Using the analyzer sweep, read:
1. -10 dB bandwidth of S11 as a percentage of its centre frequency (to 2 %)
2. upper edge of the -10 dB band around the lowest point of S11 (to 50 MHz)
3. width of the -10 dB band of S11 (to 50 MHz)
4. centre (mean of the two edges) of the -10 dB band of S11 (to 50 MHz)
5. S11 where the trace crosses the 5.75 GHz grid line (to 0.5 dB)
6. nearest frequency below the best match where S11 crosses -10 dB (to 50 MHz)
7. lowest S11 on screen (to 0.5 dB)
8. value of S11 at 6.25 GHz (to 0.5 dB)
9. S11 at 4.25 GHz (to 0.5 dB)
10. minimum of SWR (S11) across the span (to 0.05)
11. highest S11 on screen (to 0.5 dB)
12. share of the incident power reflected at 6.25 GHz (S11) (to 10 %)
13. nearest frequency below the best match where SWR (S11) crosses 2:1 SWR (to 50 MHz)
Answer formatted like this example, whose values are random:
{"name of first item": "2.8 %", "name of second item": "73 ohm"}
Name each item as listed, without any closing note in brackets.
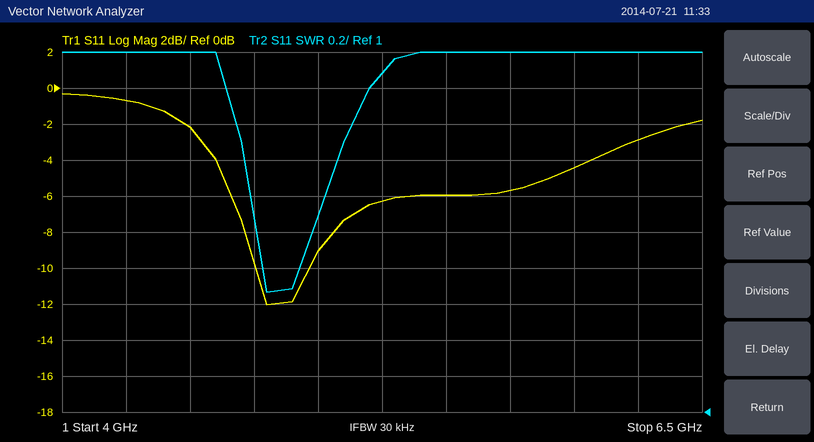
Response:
{"-10 dB bandwidth of S11 as a percentage of its centre frequency": "4 %", "upper edge of the -10 dB band around the lowest point of S11": "4.95 GHz", "width of the -10 dB band of S11": "200 MHz", "centre (mean of the two edges) of the -10 dB band of S11": "4.85 GHz", "S11 where the trace crosses the 5.75 GHz grid line": "-5.5 dB", "nearest frequency below the best match where S11 crosses -10 dB": "4.75 GHz", "lowest S11 on screen": "-12.0 dB", "value of S11 at 6.25 GHz": "-3.0 dB", "S11 at 4.25 GHz": "-0.5 dB", "minimum of SWR (S11) across the span": "1.65", "highest S11 on screen": "-0.5 dB", "share of the incident power reflected at 6.25 GHz (S11)": "50 %", "nearest frequency below the best match where SWR (S11) crosses 2:1 SWR": "4.75 GHz"}
